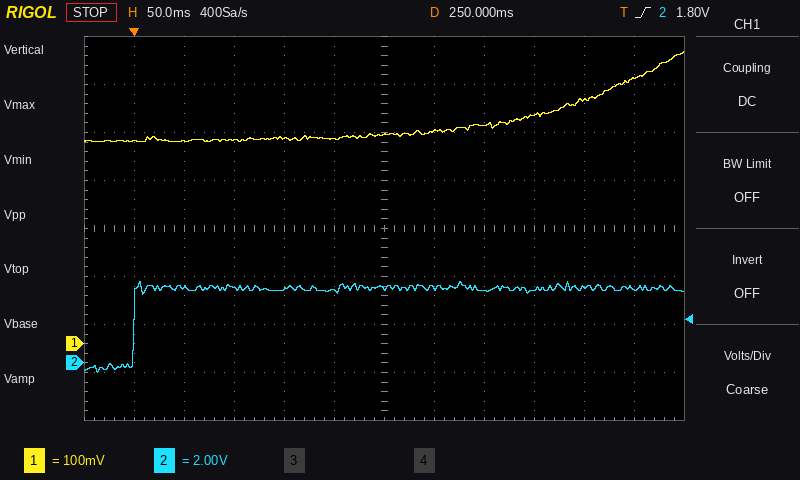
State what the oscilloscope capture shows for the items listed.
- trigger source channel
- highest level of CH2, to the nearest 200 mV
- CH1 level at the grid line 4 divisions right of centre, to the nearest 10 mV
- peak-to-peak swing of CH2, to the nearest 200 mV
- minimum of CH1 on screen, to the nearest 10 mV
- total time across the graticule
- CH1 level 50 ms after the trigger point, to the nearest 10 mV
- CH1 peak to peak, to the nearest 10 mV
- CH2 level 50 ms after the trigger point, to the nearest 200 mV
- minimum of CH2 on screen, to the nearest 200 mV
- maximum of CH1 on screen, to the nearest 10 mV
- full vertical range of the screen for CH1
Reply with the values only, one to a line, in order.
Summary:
CH2
3.4 V
510 mV
3.8 V
420 mV
600 ms
420 mV
190 mV
3.2 V
-400 mV
610 mV
800 mV
